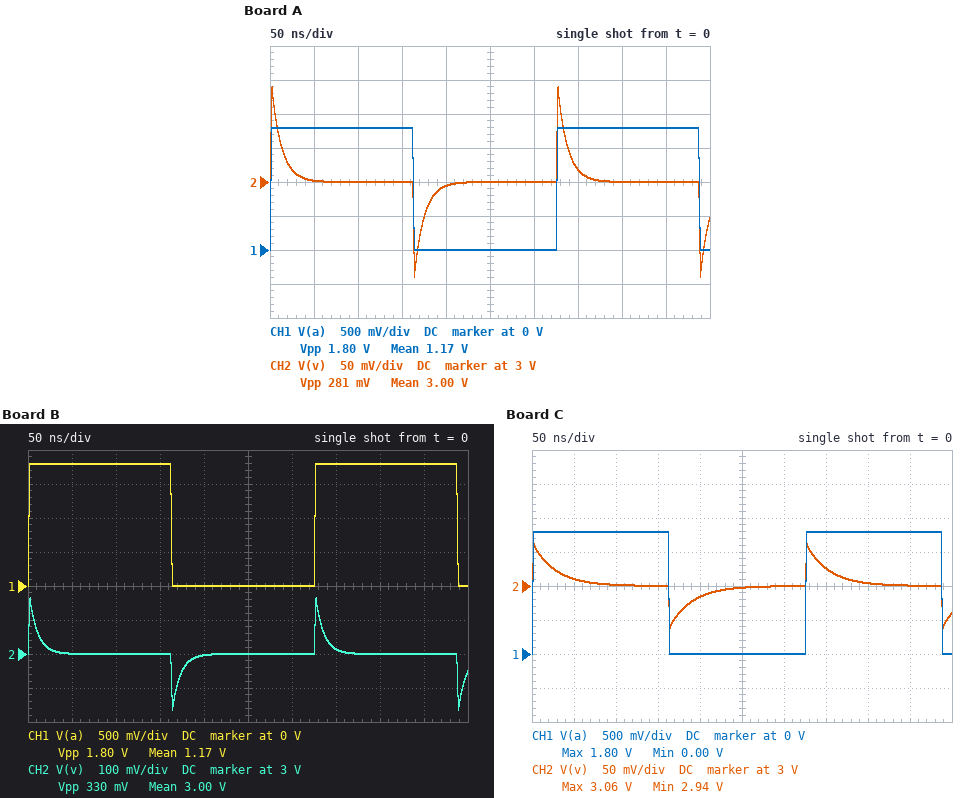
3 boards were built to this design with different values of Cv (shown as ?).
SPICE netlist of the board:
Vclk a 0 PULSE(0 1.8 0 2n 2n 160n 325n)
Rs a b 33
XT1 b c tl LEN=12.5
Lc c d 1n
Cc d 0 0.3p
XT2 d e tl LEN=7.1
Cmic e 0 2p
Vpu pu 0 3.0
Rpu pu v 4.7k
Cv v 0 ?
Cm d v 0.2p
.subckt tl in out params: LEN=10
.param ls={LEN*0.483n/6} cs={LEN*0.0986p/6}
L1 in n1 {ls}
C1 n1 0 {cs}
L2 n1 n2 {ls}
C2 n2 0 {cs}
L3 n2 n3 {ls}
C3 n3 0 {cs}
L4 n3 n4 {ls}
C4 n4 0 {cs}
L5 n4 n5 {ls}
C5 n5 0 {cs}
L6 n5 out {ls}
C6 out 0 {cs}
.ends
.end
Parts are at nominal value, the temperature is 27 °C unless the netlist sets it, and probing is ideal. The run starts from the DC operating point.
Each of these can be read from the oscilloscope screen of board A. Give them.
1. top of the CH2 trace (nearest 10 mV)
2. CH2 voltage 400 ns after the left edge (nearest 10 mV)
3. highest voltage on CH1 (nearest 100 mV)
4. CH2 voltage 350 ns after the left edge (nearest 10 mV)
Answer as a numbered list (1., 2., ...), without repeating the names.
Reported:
1. 3.14 V
2. 3.00 V
3. 1.8 V
4. 3.02 V
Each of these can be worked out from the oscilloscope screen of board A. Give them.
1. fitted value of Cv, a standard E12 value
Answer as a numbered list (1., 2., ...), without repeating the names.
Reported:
1. 2.2 pF
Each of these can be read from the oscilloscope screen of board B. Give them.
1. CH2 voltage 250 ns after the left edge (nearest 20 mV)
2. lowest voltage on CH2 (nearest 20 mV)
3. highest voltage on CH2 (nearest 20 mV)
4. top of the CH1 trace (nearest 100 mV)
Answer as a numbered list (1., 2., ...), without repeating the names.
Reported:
1. 3.00 V
2. 2.84 V
3. 3.16 V
4. 1.8 V
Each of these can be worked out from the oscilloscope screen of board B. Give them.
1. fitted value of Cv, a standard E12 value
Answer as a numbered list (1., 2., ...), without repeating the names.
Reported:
1. 1.8 pF
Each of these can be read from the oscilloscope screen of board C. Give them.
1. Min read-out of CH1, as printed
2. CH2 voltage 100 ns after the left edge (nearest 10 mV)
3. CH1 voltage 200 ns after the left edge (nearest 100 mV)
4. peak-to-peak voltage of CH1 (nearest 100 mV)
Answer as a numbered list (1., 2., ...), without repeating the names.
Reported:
1. 0.00 V
2. 3.00 V
3. 0 V
4. 1.8 V
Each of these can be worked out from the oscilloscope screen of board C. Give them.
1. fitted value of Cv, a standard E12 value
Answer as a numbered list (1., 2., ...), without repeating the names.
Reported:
1. 5.6 pF
